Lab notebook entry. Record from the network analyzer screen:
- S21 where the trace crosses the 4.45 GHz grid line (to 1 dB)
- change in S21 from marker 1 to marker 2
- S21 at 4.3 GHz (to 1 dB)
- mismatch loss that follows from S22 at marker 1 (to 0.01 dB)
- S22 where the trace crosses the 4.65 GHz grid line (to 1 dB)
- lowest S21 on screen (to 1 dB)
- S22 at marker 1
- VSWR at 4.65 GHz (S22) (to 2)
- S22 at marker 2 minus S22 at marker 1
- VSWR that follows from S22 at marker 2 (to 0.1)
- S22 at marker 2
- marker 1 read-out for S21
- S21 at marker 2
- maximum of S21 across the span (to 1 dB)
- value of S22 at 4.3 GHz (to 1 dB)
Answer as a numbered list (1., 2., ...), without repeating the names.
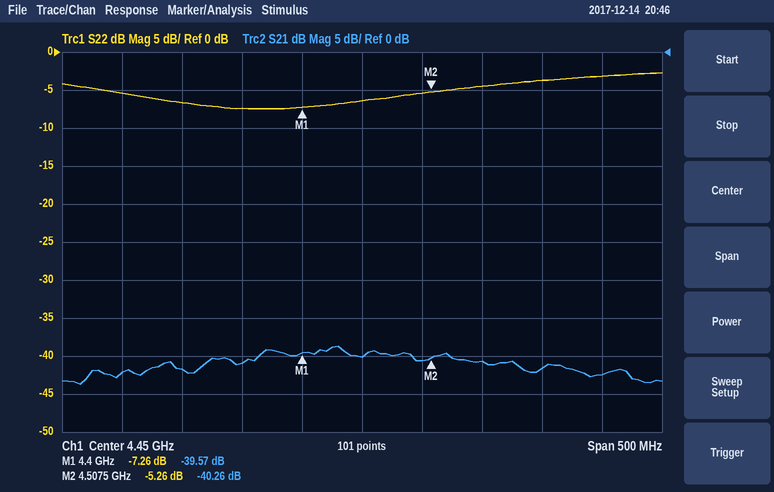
1. -40 dB
2. -0.69 dB
3. -42 dB
4. 0.90 dB
5. -3 dB
6. -44 dB
7. -7.26 dB
8. 6
9. 2.00 dB
10. 3.4
11. -5.26 dB
12. -39.57 dB
13. -40.26 dB
14. -39 dB
15. -7 dB
